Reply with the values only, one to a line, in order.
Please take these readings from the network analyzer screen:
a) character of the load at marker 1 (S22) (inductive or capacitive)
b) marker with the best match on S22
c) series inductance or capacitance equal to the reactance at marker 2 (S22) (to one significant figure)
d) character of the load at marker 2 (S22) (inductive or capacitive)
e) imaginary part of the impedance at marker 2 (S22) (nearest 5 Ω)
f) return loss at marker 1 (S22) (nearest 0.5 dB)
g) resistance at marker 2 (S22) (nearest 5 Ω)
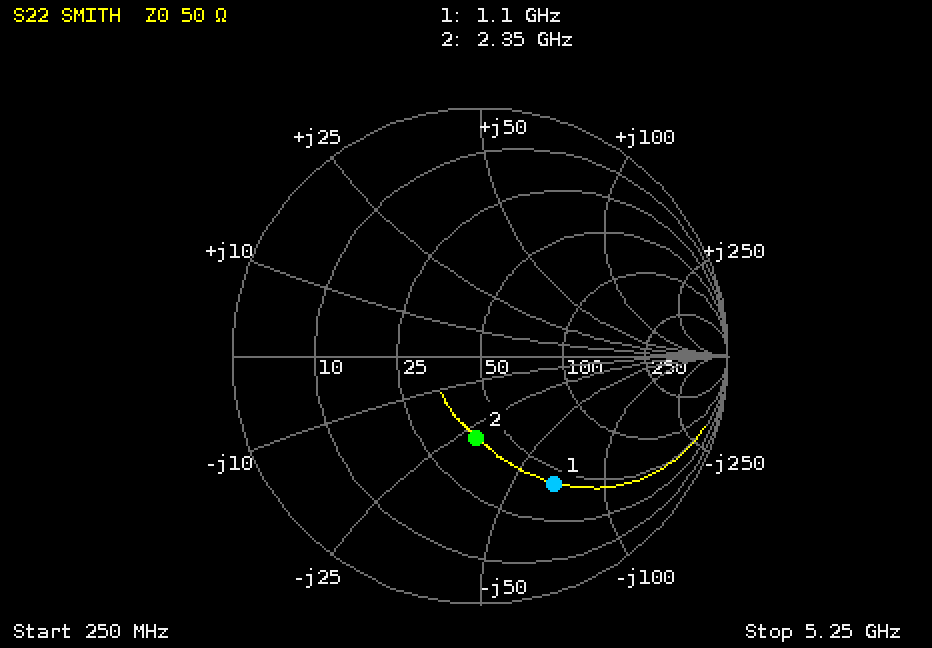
capacitive
marker 2
2 pF
capacitive
-30 Ω
4.5 dB
40 Ω
